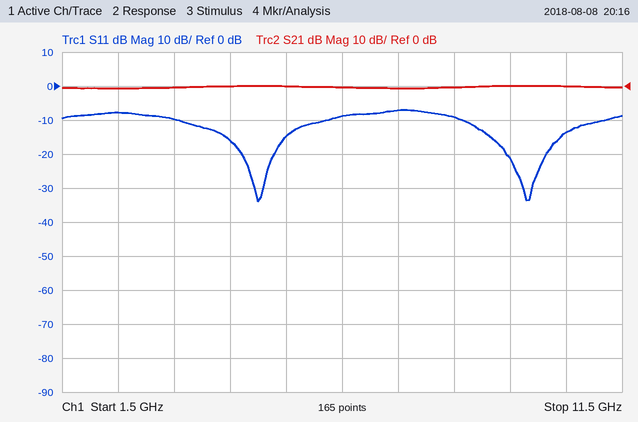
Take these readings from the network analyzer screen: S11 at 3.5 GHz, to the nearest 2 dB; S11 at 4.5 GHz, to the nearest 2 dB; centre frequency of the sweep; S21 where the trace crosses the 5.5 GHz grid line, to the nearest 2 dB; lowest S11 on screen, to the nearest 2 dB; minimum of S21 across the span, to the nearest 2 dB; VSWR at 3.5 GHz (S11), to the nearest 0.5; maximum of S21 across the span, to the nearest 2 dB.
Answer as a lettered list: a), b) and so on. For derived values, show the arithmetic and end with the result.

a) -10 dB
b) -16 dB
c) 6.5 GHz
d) 0 dB
e) -34 dB
f) 0 dB
g) |Γ| = 10^(-10/20) = 0.3162; VSWR = (1 + 0.3162)/(1 − 0.3162) ≈ 1.92, so 2.0 to the nearest 0.5
h) 0 dB
